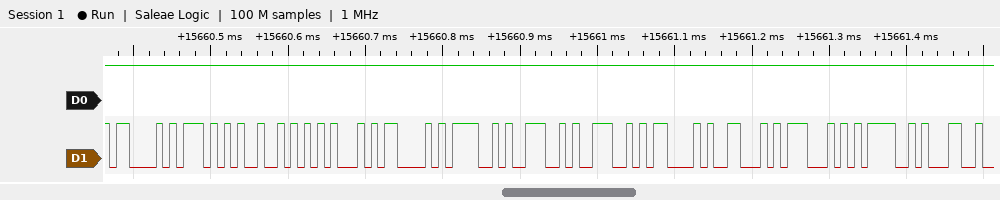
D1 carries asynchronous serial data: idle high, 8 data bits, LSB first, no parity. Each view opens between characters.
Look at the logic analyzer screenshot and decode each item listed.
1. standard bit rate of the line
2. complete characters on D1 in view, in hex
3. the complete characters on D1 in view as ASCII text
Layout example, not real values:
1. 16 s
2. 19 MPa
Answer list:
1. 115200 baud
2. 43, 57, 52, 45, 43, 4F, 4E, 4E, 43, 46, 47, 3D, 31
3. "CWRECONNCFG=1"
